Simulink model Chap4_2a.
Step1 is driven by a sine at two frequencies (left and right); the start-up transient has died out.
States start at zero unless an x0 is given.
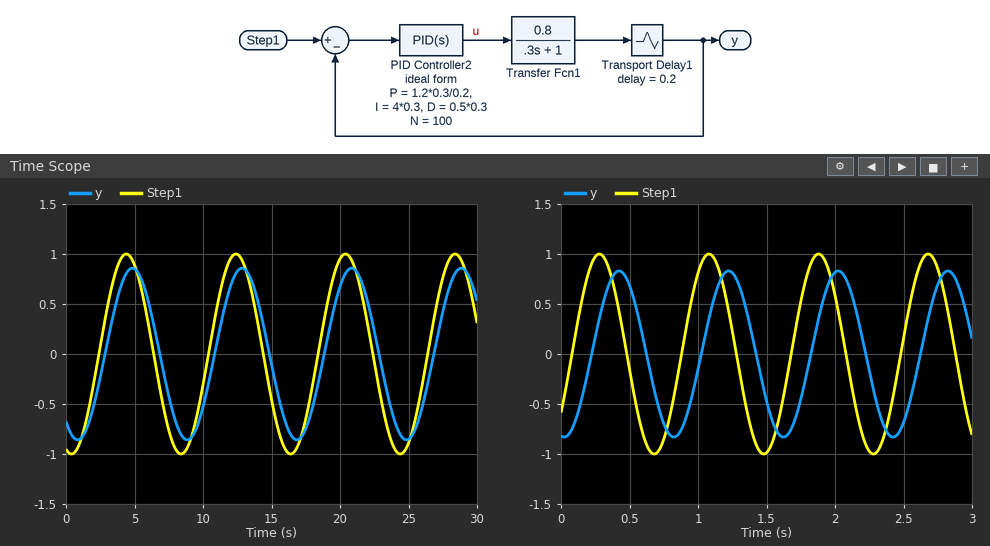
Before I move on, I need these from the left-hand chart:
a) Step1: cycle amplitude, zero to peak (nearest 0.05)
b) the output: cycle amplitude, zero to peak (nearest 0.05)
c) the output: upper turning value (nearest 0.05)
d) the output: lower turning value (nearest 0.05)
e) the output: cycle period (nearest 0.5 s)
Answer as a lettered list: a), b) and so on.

a) 1.00
b) 0.85
c) 0.85
d) -0.85
e) 8.0 s
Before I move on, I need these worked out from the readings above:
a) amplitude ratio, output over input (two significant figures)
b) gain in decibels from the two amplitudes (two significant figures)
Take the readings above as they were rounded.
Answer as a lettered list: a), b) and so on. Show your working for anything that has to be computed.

a) 0.85 / 1 = 0.85
b) 20 log10(0.85 / 1) = -1.4 dB
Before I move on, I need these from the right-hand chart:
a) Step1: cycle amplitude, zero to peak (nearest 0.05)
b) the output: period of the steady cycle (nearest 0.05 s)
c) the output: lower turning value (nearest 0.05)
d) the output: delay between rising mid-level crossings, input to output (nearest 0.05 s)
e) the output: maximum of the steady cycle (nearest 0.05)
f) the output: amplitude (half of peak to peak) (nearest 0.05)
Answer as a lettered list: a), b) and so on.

a) 1.00
b) 0.80 s
c) -0.85
d) 0.15 s
e) 0.85
f) 0.85
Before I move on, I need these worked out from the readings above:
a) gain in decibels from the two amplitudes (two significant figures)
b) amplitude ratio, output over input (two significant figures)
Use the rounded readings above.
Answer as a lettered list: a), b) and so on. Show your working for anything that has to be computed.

a) 20 log10(0.85 / 1) = -1.4 dB
b) 0.85 / 1 = 0.85
